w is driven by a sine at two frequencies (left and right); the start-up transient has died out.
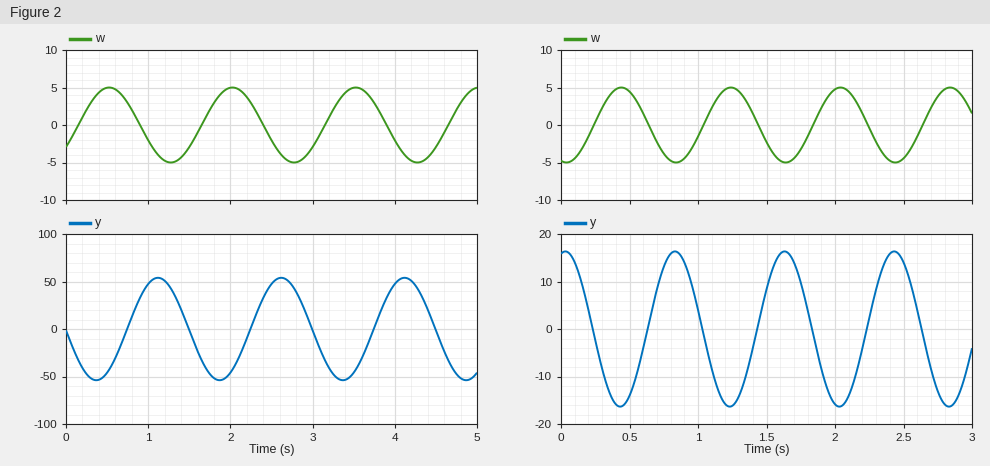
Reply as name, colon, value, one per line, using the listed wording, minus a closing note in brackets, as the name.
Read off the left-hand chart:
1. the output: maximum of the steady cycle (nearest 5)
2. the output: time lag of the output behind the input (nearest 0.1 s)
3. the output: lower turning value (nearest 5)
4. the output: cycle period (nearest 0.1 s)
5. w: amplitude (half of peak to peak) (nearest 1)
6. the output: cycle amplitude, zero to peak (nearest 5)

the output: maximum of the steady cycle: 55
the output: time lag of the output behind the input: 0.6 s
the output: lower turning value: -55
the output: cycle period: 1.5 s
w: amplitude (half of peak to peak): 5
the output: cycle amplitude, zero to peak: 55
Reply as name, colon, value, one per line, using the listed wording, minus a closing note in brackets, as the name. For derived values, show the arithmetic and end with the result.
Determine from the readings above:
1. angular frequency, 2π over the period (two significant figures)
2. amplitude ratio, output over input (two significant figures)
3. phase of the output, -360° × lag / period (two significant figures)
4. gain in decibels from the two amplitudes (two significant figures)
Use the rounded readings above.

angular frequency, 2π over the period: 2π / 1.5 = 4.2 rad/s
amplitude ratio, output over input: 55 / 5 = 11
phase of the output, -360° × lag / period: -360 × 0.6 / 1.5 = -140°
gain in decibels from the two amplitudes: 20 log10(55 / 5) = 21 dB
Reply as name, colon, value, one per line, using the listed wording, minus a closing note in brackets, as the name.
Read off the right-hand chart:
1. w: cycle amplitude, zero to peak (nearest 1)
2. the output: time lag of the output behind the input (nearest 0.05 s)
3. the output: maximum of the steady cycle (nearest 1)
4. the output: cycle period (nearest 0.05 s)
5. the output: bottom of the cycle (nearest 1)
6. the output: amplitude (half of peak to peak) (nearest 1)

w: cycle amplitude, zero to peak: 5
the output: time lag of the output behind the input: 0.40 s
the output: maximum of the steady cycle: 16
the output: cycle period: 0.80 s
the output: bottom of the cycle: -16
the output: amplitude (half of peak to peak): 16
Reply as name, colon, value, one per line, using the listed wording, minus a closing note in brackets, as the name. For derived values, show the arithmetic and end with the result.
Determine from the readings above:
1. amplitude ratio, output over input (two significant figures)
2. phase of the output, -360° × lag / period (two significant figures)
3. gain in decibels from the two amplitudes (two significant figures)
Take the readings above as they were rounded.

amplitude ratio, output over input: 16 / 5 = 3.2
phase of the output, -360° × lag / period: -360 × 0.4 / 0.8 = -180°
gain in decibels from the two amplitudes: 20 log10(16 / 5) = 10 dB
